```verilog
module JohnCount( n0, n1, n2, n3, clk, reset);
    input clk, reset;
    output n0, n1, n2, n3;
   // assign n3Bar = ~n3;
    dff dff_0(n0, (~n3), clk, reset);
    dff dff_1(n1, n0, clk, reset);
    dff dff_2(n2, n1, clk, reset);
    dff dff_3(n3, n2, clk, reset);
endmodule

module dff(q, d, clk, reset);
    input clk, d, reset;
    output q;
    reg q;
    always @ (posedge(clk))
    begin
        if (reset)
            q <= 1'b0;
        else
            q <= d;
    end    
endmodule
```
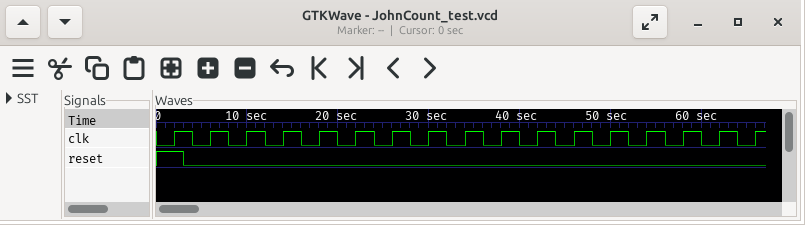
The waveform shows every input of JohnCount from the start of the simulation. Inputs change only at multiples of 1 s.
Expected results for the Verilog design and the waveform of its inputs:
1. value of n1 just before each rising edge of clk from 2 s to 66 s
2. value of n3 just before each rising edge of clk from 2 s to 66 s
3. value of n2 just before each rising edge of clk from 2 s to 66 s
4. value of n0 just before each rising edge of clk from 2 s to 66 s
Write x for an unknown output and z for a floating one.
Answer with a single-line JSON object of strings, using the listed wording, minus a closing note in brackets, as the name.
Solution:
{"value of n1 just before each rising edge of clk from 2 s to 66 s": "x 0 0 1 1 1 1 0 0 0 0 1 1 1 1 0 0", "value of n3 just before each rising edge of clk from 2 s to 66 s": "x 0 0 0 0 1 1 1 1 0 0 0 0 1 1 1 1", "value of n2 just before each rising edge of clk from 2 s to 66 s": "x 0 0 0 1 1 1 1 0 0 0 0 1 1 1 1 0", "value of n0 just before each rising edge of clk from 2 s to 66 s": "x 0 1 1 1 1 0 0 0 0 1 1 1 1 0 0 0"}
